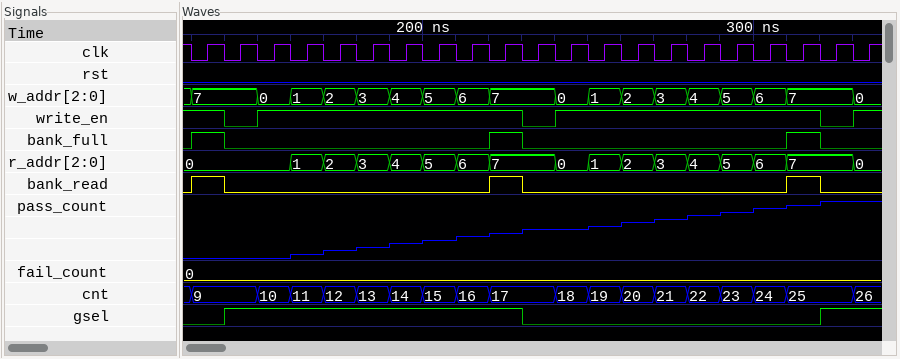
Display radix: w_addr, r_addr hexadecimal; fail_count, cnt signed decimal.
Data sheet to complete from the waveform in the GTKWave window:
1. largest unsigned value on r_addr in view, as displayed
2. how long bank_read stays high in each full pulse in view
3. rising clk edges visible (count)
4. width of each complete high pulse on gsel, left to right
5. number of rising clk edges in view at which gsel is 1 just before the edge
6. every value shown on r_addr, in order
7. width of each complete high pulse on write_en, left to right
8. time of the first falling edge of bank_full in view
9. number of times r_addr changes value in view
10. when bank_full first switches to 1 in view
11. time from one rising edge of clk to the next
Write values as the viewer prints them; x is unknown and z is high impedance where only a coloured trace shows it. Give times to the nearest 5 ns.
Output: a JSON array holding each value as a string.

["7", "10 ns, 10 ns, 10 ns", "21", "90 ns", "11", "0, 1, 2, 3, 4, 5, 6, 7, 0, 1, 2, 3, 4, 5, 6, 7, 0", "80 ns, 80 ns", "140 ns", "16", "130 ns", "10 ns"]
